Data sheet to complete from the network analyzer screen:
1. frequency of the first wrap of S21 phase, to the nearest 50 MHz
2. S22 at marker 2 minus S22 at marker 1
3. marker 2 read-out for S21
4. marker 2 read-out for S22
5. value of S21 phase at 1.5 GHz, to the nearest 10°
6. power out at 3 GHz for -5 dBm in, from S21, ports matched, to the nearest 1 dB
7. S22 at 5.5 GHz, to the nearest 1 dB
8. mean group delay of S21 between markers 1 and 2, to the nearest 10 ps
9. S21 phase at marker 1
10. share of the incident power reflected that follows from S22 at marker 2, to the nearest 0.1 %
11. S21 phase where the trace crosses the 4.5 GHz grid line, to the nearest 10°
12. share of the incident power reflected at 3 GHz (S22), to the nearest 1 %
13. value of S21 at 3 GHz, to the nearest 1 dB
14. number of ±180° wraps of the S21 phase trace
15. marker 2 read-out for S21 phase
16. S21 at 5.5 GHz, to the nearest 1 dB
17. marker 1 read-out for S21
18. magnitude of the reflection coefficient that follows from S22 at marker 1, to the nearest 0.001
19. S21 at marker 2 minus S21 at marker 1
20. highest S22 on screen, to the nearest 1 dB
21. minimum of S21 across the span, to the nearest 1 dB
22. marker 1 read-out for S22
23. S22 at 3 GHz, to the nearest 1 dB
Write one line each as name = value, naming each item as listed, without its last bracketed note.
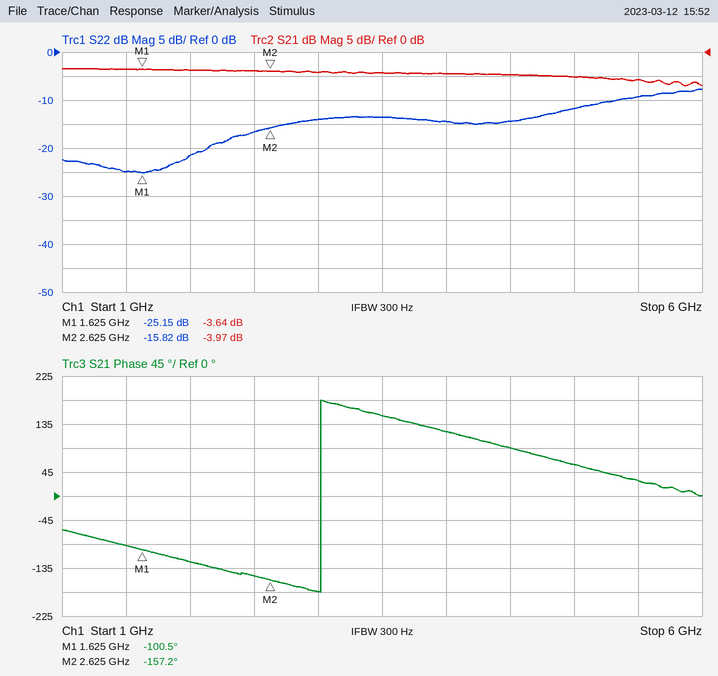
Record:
frequency of the first wrap of S21 phase, to the nearest 50 MHz = 3.00 GHz
S22 at marker 2 minus S22 at marker 1 = 9.33 dB
marker 2 read-out for S21 = -3.97 dB
marker 2 read-out for S22 = -15.82 dB
value of S21 phase at 1.5 GHz, to the nearest 10° = -90°
power out at 3 GHz for -5 dBm in, from S21, ports matched, to the nearest 1 dB = -9 dBm
S22 at 5.5 GHz, to the nearest 1 dB = -9 dB
mean group delay of S21 between markers 1 and 2, to the nearest 10 ps = 160 ps
S21 phase at marker 1 = -100.5°
share of the incident power reflected that follows from S22 at marker 2, to the nearest 0.1 % = 2.6 %
S21 phase where the trace crosses the 4.5 GHz grid line, to the nearest 10° = 90°
share of the incident power reflected at 3 GHz (S22), to the nearest 1 % = 4 %
value of S21 at 3 GHz, to the nearest 1 dB = -4 dB
number of ±180° wraps of the S21 phase trace = 1
marker 2 read-out for S21 phase = -157.2°
S21 at 5.5 GHz, to the nearest 1 dB = -6 dB
marker 1 read-out for S21 = -3.64 dB
magnitude of the reflection coefficient that follows from S22 at marker 1, to the nearest 0.001 = 0.055
S21 at marker 2 minus S21 at marker 1 = -0.33 dB
highest S22 on screen, to the nearest 1 dB = -8 dB
minimum of S21 across the span, to the nearest 1 dB = -7 dB
marker 1 read-out for S22 = -25.15 dB
S22 at 3 GHz, to the nearest 1 dB = -14 dB
